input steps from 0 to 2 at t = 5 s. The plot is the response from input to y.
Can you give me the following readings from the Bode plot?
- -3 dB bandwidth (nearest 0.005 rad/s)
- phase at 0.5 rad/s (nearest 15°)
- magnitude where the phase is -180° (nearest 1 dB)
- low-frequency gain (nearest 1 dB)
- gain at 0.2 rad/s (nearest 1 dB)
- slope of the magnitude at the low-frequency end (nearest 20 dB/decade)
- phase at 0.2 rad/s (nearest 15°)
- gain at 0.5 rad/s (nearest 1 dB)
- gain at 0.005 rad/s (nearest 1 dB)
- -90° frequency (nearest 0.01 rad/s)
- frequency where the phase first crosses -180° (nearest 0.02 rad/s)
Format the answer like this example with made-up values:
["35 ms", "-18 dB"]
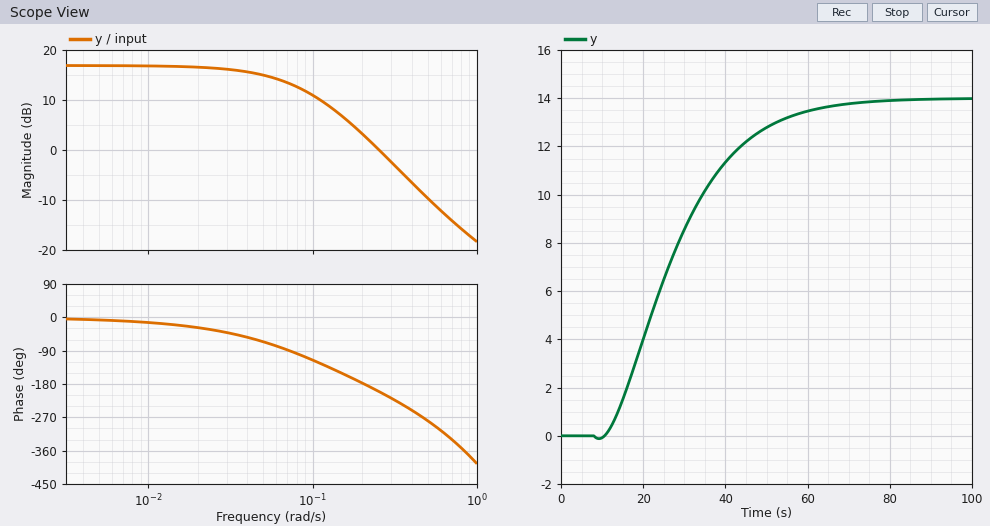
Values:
["0.065 rad/s", "-285°", "3 dB", "17 dB", "3 dB", "0 dB/decade", "-180°", "-10 dB", "17 dB", "0.07 rad/s", "0.20 rad/s"]
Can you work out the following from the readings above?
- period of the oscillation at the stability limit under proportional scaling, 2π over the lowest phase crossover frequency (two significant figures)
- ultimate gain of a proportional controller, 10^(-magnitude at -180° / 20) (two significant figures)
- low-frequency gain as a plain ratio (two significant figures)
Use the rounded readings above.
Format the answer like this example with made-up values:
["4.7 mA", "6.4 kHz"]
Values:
["31 s", "0.71", "7.1"]
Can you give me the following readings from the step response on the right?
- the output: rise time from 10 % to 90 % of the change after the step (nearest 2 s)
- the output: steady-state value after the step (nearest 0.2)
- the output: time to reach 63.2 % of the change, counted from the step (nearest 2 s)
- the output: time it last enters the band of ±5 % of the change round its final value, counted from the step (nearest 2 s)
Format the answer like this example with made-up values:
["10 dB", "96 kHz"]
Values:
["34 s", "14.0", "26 s", "52 s"]
